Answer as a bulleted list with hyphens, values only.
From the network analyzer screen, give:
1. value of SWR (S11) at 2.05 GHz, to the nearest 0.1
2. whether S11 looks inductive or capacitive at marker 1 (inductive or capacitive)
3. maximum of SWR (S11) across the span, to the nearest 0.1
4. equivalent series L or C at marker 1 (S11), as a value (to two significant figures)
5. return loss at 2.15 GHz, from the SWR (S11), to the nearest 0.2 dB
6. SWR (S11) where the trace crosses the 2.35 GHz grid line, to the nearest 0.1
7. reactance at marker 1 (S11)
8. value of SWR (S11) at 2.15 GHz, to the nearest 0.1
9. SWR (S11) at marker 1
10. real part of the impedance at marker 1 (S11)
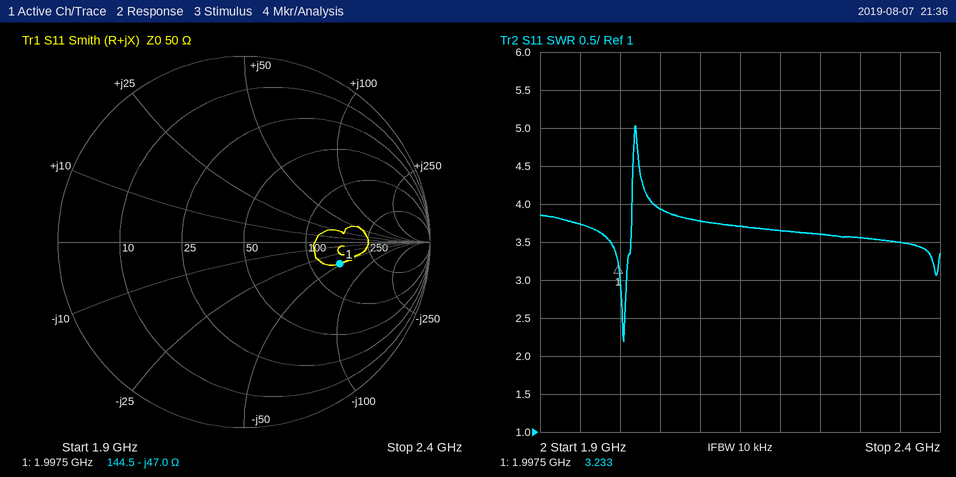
- 3.9
- capacitive
- 5.0
- 1.7 pF
- 4.8 dB
- 3.5
- -47.0 Ω
- 3.7
- 3.233
- 144.5 Ω
